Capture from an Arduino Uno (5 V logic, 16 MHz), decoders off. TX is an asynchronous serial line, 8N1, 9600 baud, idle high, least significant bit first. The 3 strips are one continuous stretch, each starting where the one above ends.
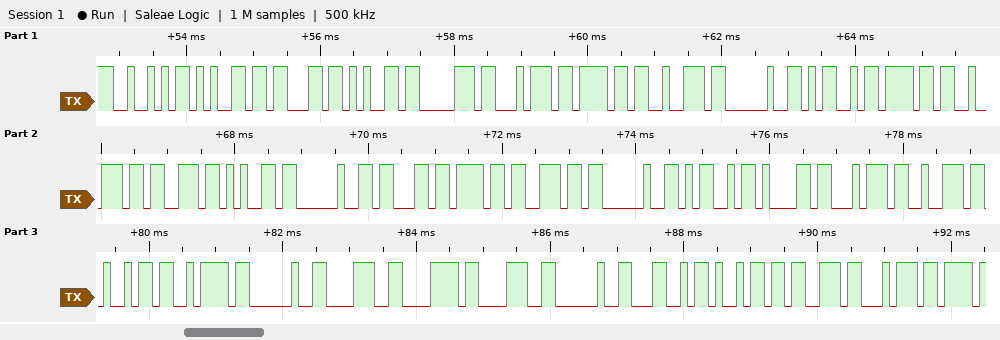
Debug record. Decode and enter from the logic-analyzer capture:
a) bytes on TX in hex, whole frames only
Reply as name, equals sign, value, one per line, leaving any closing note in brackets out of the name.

bytes on TX in hex, whole frames only = 52 65 63 65 70 74 6F 72 20 4D 6F 72 73 65 20 63 6F 6E 20 4D 61 74 72 69 7A 20 38 78 38 20 4C 69 73 74
